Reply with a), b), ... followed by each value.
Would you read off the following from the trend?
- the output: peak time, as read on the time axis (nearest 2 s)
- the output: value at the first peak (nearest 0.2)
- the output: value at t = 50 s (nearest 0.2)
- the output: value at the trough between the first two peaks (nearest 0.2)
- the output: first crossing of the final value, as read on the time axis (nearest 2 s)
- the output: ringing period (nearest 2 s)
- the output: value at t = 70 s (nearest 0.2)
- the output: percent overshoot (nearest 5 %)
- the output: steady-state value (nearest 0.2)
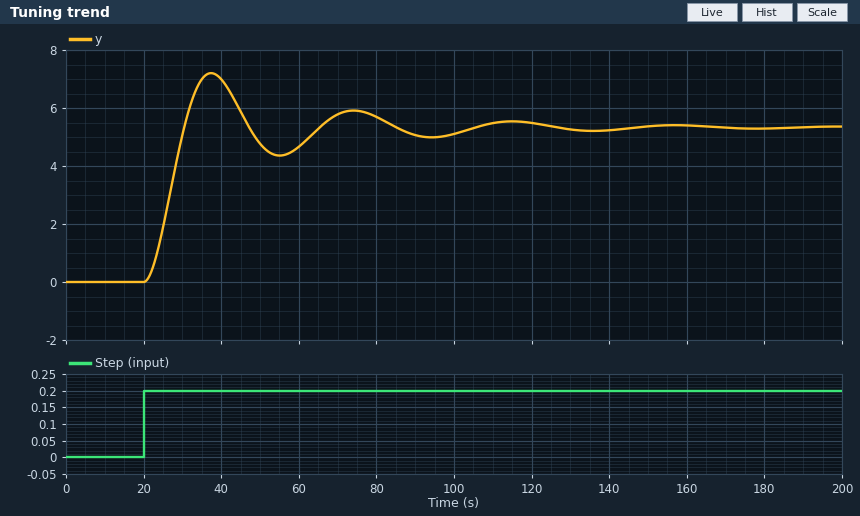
a) 38 s
b) 7.2
c) 4.8
d) 4.4
e) 30 s
f) 36 s
g) 5.8
h) 35 %
i) 5.4
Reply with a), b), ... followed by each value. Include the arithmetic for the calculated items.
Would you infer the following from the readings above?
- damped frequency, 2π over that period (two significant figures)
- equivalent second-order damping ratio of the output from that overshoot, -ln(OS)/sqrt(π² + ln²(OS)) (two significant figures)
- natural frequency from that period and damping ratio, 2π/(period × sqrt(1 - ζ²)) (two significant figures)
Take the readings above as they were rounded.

a) 2π / 36 = 0.17 rad/s
b) ln(0.35) = -1.050; 1.050 / sqrt(9.870 + 1.102) = 0.32
c) 2π / (36 × sqrt(1 - 0.32²)) = 0.18 rad/s
